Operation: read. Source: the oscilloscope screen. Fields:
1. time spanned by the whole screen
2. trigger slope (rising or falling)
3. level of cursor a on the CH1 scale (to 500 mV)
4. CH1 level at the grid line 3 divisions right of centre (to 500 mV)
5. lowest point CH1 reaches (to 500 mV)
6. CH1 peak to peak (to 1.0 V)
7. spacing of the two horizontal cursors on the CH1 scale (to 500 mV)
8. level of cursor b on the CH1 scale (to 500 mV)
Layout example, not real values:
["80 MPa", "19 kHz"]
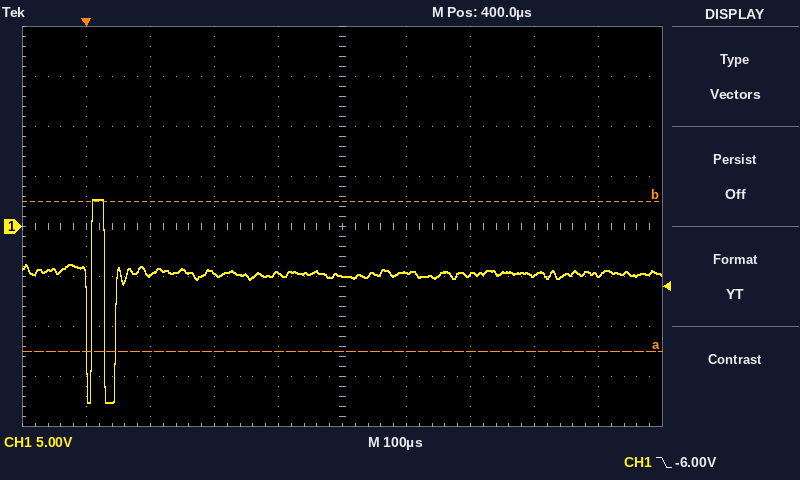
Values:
["1 ms", "falling", "-12.5 V", "-5.0 V", "-17.5 V", "20.0 V", "15.0 V", "2.5 V"]
